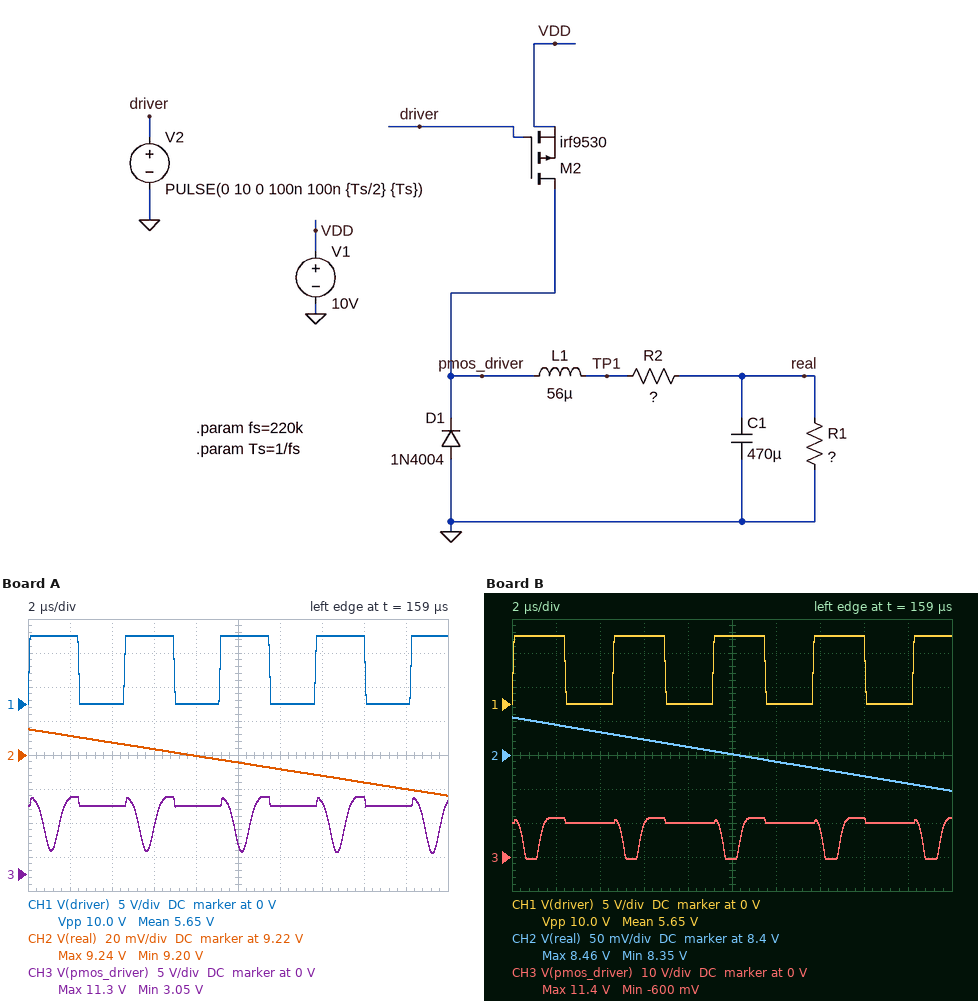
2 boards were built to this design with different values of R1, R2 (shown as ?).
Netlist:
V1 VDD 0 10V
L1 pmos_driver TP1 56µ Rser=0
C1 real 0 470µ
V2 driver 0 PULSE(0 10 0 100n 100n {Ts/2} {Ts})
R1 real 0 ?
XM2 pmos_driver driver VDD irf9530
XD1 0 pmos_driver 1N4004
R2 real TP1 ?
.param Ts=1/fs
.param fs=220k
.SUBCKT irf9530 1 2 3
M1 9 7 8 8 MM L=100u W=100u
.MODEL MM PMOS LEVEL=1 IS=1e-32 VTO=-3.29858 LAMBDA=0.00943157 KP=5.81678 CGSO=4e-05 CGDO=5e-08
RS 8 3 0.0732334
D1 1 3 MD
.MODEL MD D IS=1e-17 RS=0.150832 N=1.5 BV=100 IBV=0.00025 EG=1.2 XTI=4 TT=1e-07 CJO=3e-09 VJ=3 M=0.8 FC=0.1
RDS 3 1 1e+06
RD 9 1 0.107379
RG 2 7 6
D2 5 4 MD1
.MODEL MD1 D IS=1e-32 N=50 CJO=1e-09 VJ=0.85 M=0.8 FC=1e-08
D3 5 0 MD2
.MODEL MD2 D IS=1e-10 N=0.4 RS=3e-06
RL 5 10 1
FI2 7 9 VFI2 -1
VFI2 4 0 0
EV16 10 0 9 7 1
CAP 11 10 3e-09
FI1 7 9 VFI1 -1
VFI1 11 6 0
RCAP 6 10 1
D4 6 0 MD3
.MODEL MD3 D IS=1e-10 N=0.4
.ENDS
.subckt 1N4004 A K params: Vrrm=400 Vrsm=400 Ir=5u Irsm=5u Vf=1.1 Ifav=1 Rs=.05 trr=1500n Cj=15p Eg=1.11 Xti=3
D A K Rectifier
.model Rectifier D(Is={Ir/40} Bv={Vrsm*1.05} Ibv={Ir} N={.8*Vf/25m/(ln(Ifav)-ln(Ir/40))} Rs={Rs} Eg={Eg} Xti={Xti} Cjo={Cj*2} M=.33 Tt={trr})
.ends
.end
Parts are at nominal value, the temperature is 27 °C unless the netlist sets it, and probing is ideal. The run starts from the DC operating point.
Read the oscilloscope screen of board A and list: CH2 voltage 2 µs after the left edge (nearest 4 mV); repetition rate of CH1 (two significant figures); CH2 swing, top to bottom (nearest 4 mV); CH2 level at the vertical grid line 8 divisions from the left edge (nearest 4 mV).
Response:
9.232 V
220 kHz
40 mV
9.204 V
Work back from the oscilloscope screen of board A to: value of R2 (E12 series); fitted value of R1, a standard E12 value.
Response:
0.27 Ω
10 Ω
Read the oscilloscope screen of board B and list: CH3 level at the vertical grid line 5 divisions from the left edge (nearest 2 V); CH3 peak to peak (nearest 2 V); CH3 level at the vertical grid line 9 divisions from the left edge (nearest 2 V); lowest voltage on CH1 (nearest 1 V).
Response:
0 V
12 V
10 V
0 V
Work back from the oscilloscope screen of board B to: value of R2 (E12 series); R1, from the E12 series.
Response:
0.047 Ω
3.3 Ω
